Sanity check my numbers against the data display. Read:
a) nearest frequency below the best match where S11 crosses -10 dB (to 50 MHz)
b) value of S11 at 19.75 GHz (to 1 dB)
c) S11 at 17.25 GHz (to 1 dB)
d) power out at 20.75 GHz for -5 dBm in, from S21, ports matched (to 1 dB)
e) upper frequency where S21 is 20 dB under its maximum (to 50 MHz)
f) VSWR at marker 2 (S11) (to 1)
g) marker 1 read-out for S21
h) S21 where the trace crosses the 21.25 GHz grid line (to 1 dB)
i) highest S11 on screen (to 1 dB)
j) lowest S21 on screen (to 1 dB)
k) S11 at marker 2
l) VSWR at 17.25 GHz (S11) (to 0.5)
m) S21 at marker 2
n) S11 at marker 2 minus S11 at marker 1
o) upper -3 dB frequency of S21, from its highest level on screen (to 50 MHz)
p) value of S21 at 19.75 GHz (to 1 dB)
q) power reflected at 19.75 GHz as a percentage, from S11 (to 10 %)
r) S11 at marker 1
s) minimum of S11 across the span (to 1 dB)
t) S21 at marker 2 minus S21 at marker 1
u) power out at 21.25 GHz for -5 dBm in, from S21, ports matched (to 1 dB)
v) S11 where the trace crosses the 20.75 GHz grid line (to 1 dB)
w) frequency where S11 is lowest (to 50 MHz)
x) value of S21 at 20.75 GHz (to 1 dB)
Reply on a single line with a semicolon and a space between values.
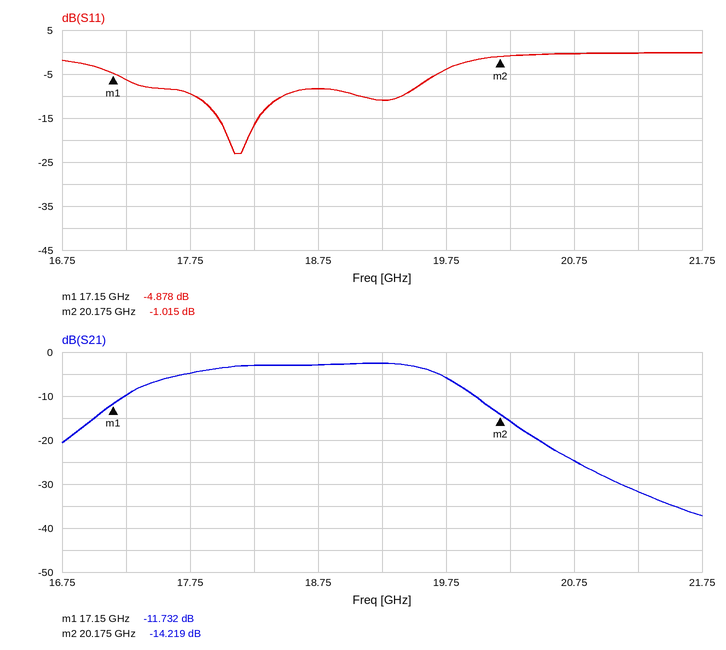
17.80 GHz; -4 dB; -6 dB; -30 dBm; 20.60 GHz; 17; -11.732 dB; -32 dB; 0 dB; -37 dB; -1.015 dB; 3.0; -14.219 dB; 3.863 dB; 19.75 GHz; -6 dB; 40 %; -4.878 dB; -23 dB; -2.487 dB; -37 dBm; 0 dB; 18.10 GHz; -25 dB
